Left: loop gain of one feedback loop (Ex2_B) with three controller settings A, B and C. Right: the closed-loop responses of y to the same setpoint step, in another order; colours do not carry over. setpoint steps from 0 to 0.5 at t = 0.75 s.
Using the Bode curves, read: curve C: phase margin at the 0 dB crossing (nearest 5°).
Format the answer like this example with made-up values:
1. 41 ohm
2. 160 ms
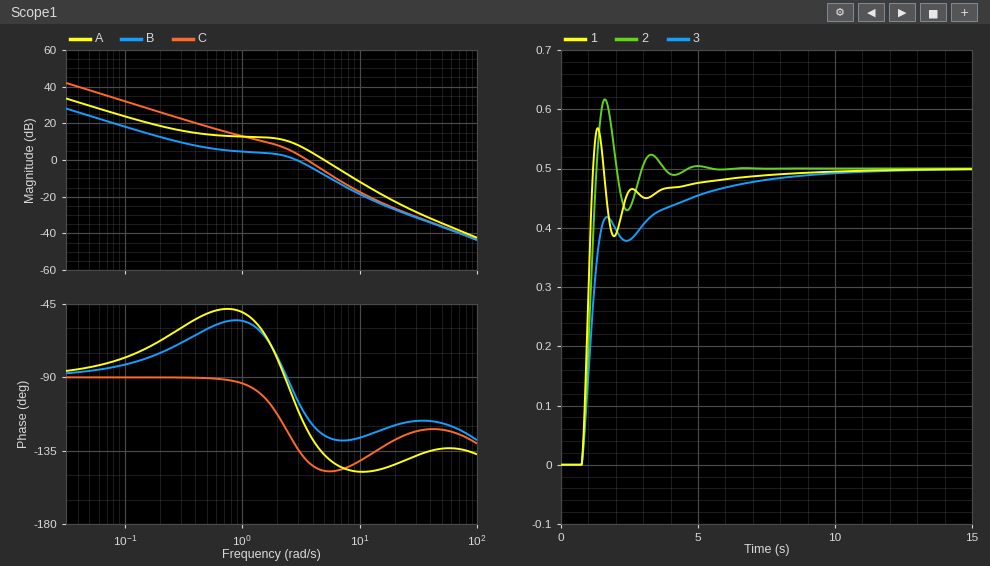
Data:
1. 40°
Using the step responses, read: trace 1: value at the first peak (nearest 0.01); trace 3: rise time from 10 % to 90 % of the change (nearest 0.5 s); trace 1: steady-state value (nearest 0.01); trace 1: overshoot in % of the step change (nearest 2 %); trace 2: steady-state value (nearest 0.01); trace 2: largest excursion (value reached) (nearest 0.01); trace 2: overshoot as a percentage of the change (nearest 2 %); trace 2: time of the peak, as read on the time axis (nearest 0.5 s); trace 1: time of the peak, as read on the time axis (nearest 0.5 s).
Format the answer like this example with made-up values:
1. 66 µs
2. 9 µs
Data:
1. 0.57
2. 4.0 s
3. 0.50
4. 14 %
5. 0.50
6. 0.62
7. 24 %
8. 1.5 s
9. 1.5 s
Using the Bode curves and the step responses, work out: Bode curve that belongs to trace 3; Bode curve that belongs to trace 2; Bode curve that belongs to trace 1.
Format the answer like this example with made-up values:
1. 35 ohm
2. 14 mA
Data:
1. B
2. C
3. A
